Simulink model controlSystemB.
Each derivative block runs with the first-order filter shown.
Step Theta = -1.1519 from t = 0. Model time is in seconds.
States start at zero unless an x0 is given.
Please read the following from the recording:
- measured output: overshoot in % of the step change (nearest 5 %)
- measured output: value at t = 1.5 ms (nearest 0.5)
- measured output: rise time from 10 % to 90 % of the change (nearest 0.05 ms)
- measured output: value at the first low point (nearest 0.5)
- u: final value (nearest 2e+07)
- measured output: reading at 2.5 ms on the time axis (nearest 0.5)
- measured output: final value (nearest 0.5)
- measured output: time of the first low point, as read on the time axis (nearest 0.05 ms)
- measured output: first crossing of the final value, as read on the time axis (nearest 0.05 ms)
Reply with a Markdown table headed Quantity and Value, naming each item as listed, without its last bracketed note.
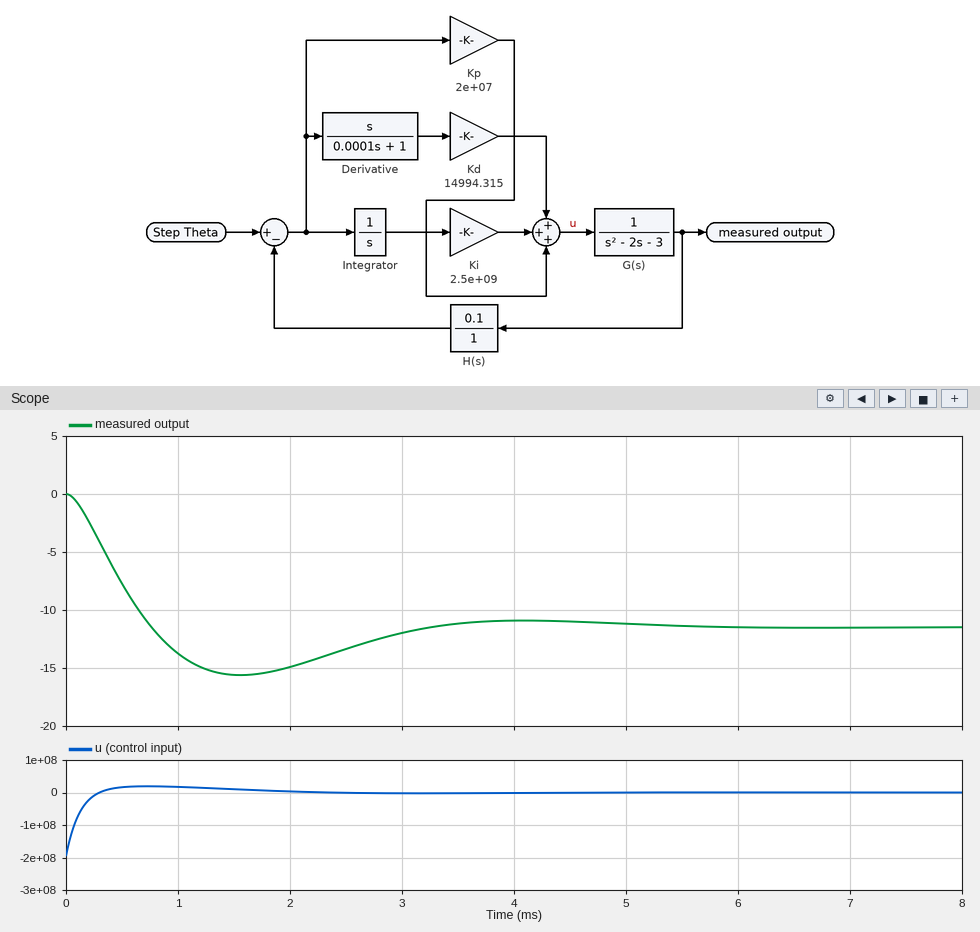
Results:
| Quantity | Value |
|---|---|
| measured output: overshoot in % of the step change | 35 % |
| measured output: value at t = 1.5 ms | -15.5 |
| measured output: rise time from 10 % to 90 % of the change | 0.55 ms |
| measured output: value at the first low point | -15.5 |
| u: final value | 0 |
| measured output: reading at 2.5 ms on the time axis | -13.5 |
| measured output: final value | -11.5 |
| measured output: time of the first low point, as read on the time axis | 1.55 ms |
| measured output: first crossing of the final value, as read on the time axis | 0.75 ms |
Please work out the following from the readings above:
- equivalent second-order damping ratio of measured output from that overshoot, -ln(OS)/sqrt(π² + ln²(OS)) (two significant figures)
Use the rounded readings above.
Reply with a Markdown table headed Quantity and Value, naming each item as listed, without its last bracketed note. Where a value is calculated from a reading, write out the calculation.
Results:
| Quantity | Value |
|---|---|
| equivalent second-order damping ratio of measured output from that overshoot, -ln(OS)/sqrt(π² + ln²(OS)) | ln(0.35) = -1.050; 1.050 / sqrt(9.870 + 1.102) = 0.32 |
